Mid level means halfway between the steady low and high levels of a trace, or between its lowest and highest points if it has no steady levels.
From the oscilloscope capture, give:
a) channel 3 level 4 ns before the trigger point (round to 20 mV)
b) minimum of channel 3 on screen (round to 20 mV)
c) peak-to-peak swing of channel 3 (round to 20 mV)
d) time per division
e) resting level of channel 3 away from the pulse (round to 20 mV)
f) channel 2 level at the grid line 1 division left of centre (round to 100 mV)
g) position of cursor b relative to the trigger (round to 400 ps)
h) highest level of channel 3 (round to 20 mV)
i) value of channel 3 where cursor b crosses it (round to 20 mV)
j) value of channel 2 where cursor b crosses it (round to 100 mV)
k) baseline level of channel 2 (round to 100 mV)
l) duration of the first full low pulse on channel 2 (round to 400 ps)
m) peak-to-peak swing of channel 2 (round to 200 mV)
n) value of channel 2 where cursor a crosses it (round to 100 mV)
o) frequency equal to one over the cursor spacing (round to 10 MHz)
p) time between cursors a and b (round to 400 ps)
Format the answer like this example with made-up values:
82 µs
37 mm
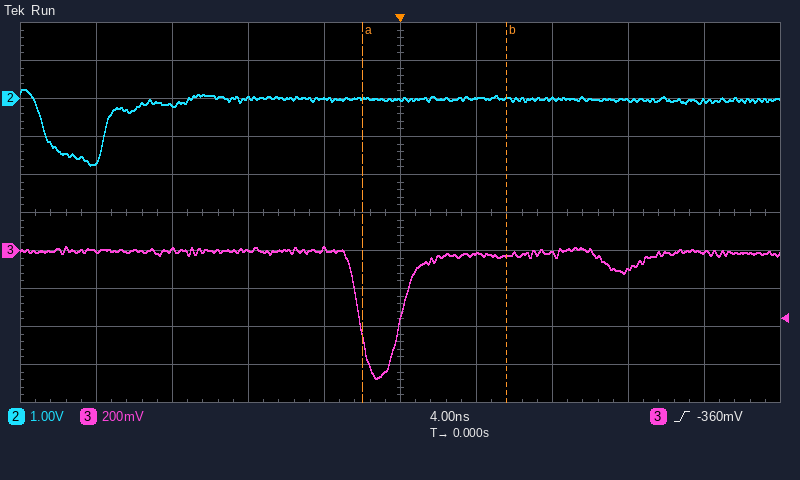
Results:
0 mV
-680 mV
700 mV
4 ns
0 mV
0.0 V
+5.6 ns
20 mV
-20 mV
0.0 V
0.0 V
3.2 ns
2.0 V
0.0 V
130 MHz
7.6 ns
